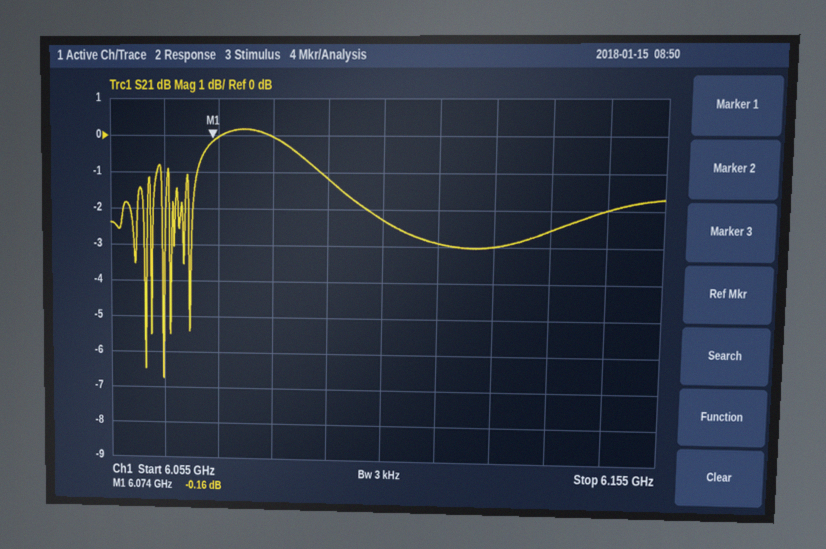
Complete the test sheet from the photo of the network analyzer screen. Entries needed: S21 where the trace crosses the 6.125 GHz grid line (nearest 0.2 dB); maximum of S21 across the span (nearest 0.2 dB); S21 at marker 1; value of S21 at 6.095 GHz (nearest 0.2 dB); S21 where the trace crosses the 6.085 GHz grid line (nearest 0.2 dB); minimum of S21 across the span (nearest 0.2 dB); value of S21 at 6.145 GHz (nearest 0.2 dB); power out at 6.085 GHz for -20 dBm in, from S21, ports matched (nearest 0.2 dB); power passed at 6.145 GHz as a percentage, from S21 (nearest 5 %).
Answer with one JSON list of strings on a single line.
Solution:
["-3.0 dB", "0.2 dB", "-0.16 dB", "-1.2 dB", "0.0 dB", "-6.8 dB", "-2.0 dB", "-20.0 dBm", "65 %"]
